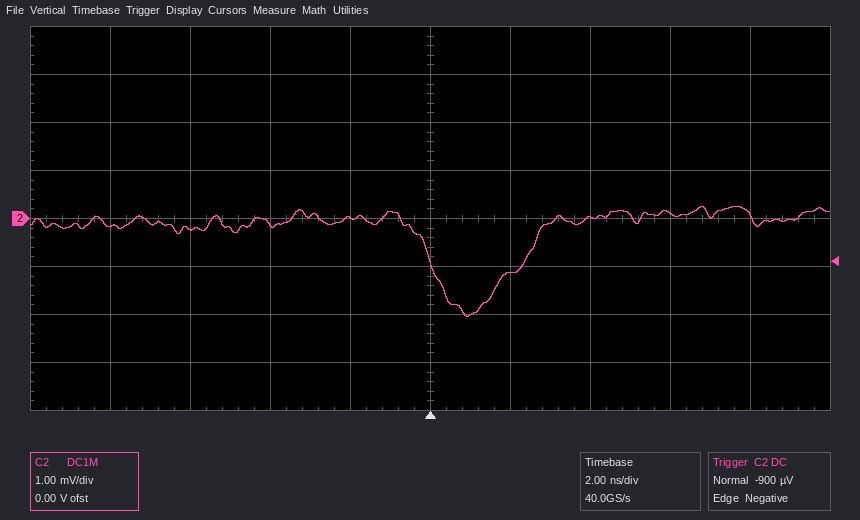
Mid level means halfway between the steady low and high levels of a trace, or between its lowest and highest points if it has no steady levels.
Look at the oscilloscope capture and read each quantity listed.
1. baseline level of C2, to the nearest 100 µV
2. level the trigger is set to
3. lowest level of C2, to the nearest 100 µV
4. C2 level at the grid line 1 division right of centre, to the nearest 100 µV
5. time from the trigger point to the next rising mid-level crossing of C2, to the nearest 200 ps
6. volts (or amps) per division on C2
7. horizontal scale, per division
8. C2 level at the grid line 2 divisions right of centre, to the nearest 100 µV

-100 µV
-900 µV
-2.0 mV
-1.1 mV
2.4 ns
1 mV
2 ns
0.0 mV
